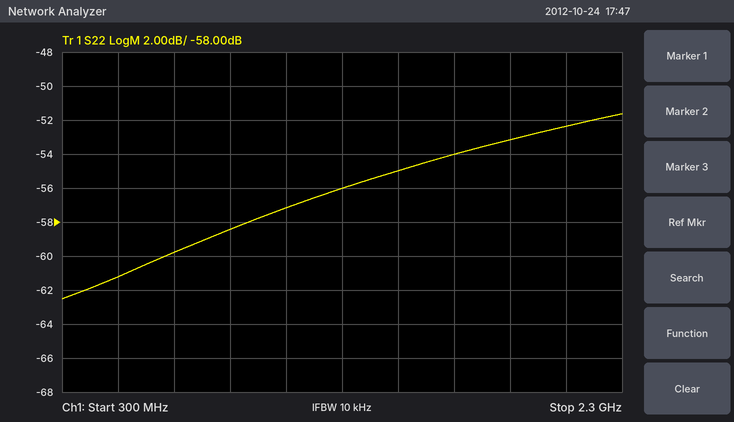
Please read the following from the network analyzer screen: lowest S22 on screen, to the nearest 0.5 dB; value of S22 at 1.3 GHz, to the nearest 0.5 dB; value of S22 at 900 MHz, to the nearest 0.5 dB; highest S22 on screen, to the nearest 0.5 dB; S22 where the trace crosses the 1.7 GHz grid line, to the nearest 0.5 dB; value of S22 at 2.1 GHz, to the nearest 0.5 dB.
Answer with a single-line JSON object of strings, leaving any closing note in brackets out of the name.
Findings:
{"lowest S22 on screen, to the nearest 0.5 dB": "-62.5 dB", "value of S22 at 1.3 GHz, to the nearest 0.5 dB": "-56.0 dB", "value of S22 at 900 MHz, to the nearest 0.5 dB": "-58.5 dB", "highest S22 on screen, to the nearest 0.5 dB": "-51.5 dB", "S22 where the trace crosses the 1.7 GHz grid line, to the nearest 0.5 dB": "-54.0 dB", "value of S22 at 2.1 GHz, to the nearest 0.5 dB": "-52.5 dB"}
